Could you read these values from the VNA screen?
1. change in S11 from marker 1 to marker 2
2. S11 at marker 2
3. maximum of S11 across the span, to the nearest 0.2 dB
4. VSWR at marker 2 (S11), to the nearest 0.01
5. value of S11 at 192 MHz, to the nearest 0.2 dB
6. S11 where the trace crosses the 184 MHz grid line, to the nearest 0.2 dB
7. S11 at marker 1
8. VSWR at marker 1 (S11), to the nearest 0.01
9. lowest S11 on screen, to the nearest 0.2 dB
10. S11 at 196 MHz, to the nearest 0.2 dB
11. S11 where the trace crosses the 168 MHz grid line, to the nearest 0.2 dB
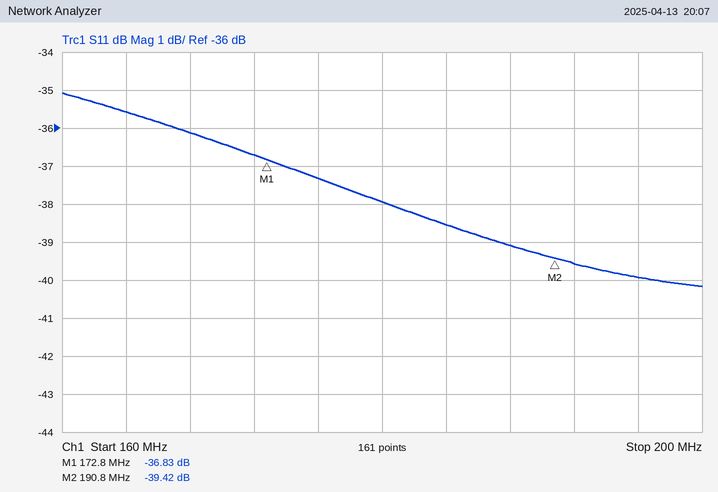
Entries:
-2.59 dB
-39.42 dB
-35.0 dB
1.02
-39.6 dB
-38.6 dB
-36.83 dB
1.03
-40.2 dB
-40.0 dB
-36.2 dB
